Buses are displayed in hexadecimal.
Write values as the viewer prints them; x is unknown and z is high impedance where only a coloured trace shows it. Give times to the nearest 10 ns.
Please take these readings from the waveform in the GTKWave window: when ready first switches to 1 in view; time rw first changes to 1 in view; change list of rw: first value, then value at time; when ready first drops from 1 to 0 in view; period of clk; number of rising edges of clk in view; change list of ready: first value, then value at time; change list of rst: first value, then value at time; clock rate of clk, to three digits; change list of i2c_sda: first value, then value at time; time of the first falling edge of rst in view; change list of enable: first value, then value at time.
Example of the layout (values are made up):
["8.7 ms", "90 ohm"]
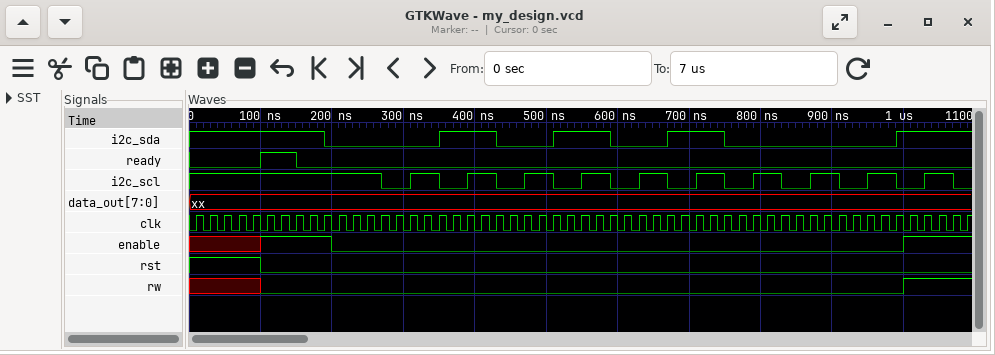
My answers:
["100 ns", "1000 ns", "x, 0 at 100 ns, 1 at 1000 ns", "150 ns", "20 ns", "55", "0, 1 at 100 ns, 0 at 150 ns", "1, 0 at 100 ns", "50.0 MHz", "1, 0 at 190 ns, 1 at 350 ns, 0 at 430 ns, 1 at 510 ns, 0 at 590 ns, 1 at 670 ns, 0 at 750 ns, 1 at 990 ns", "100 ns", "x, 1 at 100 ns, 0 at 200 ns, 1 at 1000 ns"]
